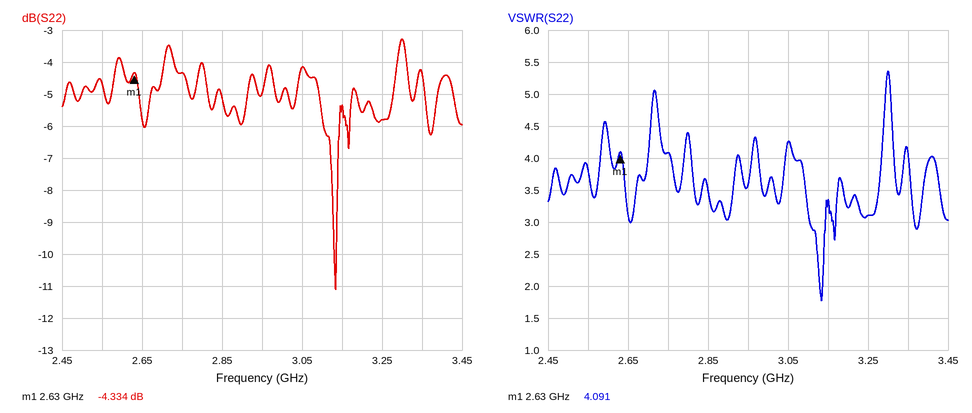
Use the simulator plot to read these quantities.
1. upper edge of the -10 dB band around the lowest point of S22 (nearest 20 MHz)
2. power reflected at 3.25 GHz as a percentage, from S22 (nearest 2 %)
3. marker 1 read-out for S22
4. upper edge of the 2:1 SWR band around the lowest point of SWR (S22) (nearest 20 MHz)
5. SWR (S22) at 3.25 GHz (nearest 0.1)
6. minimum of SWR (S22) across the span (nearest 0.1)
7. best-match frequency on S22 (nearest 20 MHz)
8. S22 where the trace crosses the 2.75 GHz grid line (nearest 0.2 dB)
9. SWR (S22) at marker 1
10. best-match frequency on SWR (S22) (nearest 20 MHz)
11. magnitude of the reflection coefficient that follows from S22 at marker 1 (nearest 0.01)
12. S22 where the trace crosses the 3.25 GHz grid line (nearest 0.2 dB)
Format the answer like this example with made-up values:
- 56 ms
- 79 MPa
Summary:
- 3.14 GHz
- 26 %
- -4.334 dB
- 3.14 GHz
- 3.1
- 1.8
- 3.14 GHz
- -4.4 dB
- 4.091
- 3.14 GHz
- 0.61
- -5.8 dB
